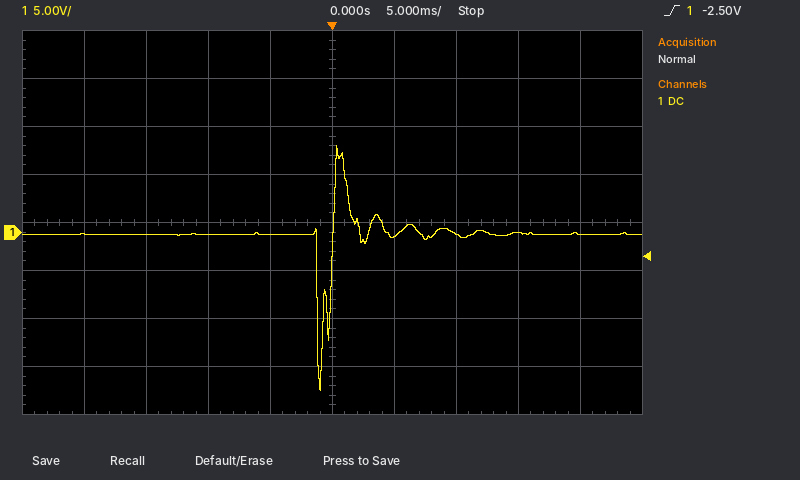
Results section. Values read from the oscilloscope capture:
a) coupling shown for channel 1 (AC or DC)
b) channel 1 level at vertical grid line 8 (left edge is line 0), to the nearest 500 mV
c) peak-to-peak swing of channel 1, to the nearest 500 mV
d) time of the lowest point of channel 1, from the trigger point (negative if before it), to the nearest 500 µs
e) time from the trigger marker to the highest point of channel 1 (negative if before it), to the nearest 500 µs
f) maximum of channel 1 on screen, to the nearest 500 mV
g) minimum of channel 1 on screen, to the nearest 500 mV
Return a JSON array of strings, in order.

["DC", "0.0 V", "25.5 V", "-1.0 ms", "+500 µs", "9.0 V", "-16.5 V"]
